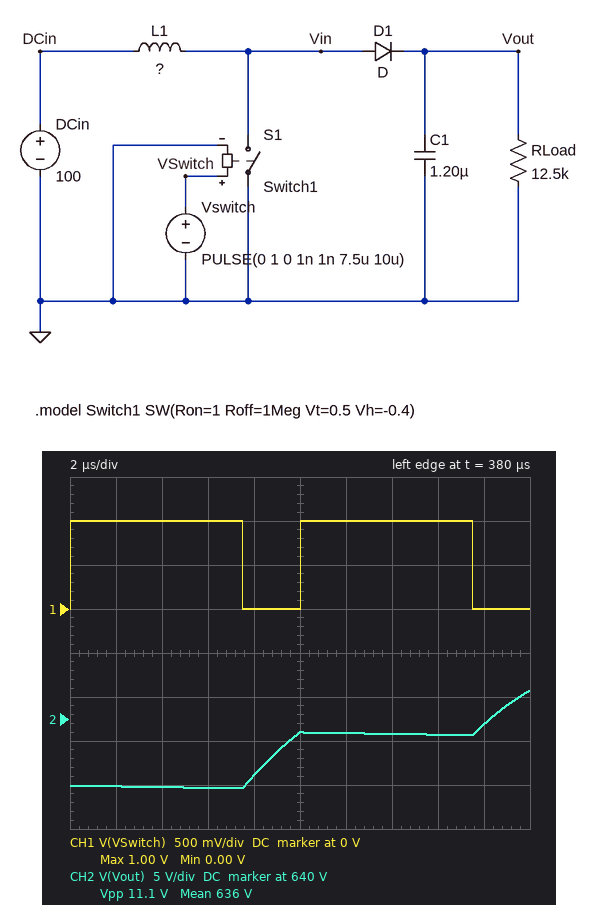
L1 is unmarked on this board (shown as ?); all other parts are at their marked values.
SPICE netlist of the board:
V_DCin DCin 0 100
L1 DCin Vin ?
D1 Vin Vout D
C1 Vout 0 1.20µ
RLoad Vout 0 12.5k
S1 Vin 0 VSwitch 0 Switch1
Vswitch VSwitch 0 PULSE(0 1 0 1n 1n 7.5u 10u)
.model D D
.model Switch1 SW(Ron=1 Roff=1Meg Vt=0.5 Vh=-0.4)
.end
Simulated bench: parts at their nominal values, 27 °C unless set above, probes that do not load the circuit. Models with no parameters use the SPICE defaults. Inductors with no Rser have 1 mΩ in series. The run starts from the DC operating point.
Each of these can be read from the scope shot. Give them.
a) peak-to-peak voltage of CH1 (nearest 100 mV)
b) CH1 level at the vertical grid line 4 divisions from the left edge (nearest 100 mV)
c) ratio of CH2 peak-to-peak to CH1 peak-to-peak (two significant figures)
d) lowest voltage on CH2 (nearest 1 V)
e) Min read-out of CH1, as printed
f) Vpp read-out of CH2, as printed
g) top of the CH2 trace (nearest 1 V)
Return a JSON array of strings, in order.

["1.0 V", "0 V", "11", "632 V", "0.00 V", "11.1 V", "643 V"]
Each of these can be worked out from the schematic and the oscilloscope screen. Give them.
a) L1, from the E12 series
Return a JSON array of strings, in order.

["1 mH"]
